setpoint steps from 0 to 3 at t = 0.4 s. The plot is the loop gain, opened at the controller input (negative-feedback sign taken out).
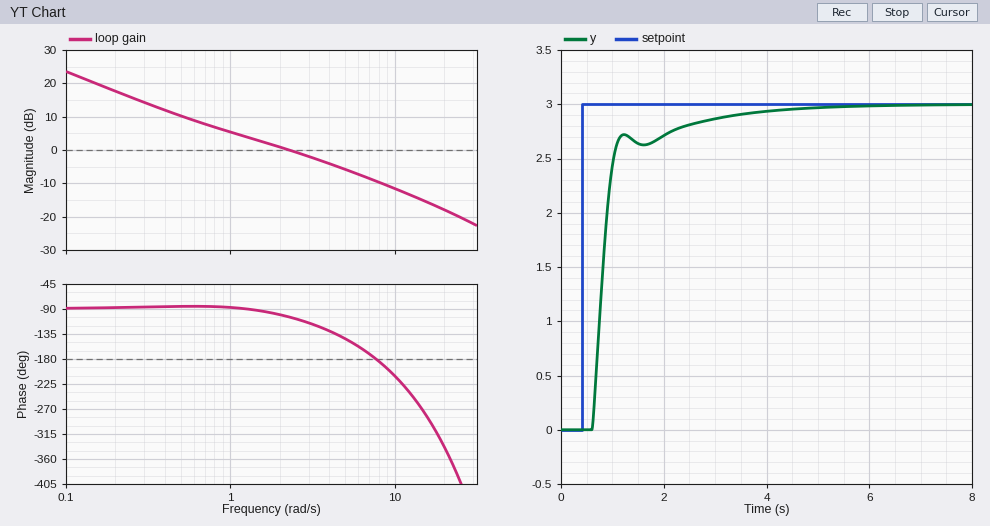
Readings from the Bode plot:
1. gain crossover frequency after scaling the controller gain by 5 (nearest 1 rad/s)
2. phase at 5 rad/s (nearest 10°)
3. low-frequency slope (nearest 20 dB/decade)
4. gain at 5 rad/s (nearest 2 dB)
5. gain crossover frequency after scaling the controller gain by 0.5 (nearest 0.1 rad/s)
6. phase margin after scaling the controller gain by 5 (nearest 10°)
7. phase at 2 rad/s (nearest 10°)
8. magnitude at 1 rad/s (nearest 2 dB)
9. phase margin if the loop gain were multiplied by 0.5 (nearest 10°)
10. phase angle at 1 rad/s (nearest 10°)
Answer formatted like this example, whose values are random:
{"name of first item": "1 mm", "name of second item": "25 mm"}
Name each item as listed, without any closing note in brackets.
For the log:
{"gain crossover frequency after scaling the controller gain by 5": "13 rad/s", "phase at 5 rad/s": "-140°", "low-frequency slope": "-20 dB/decade", "gain at 5 rad/s": "-6 dB", "gain crossover frequency after scaling the controller gain by 0.5": "0.9 rad/s", "phase margin after scaling the controller gain by 5": "-70°", "phase at 2 rad/s": "-100°", "magnitude at 1 rad/s": "6 dB", "phase margin if the loop gain were multiplied by 0.5": "90°", "phase angle at 1 rad/s": "-90°"}
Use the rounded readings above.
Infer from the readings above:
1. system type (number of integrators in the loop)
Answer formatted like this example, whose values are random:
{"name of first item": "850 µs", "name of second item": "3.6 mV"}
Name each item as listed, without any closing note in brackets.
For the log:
{"system type": "1"}
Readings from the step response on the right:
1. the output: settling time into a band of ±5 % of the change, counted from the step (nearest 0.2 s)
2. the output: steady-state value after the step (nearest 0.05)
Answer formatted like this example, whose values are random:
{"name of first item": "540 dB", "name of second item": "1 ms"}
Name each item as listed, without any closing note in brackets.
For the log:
{"the output: settling time into a band of ±5 % of the change, counted from the step": "2.4 s", "the output: steady-state value after the step": "3.00"}
